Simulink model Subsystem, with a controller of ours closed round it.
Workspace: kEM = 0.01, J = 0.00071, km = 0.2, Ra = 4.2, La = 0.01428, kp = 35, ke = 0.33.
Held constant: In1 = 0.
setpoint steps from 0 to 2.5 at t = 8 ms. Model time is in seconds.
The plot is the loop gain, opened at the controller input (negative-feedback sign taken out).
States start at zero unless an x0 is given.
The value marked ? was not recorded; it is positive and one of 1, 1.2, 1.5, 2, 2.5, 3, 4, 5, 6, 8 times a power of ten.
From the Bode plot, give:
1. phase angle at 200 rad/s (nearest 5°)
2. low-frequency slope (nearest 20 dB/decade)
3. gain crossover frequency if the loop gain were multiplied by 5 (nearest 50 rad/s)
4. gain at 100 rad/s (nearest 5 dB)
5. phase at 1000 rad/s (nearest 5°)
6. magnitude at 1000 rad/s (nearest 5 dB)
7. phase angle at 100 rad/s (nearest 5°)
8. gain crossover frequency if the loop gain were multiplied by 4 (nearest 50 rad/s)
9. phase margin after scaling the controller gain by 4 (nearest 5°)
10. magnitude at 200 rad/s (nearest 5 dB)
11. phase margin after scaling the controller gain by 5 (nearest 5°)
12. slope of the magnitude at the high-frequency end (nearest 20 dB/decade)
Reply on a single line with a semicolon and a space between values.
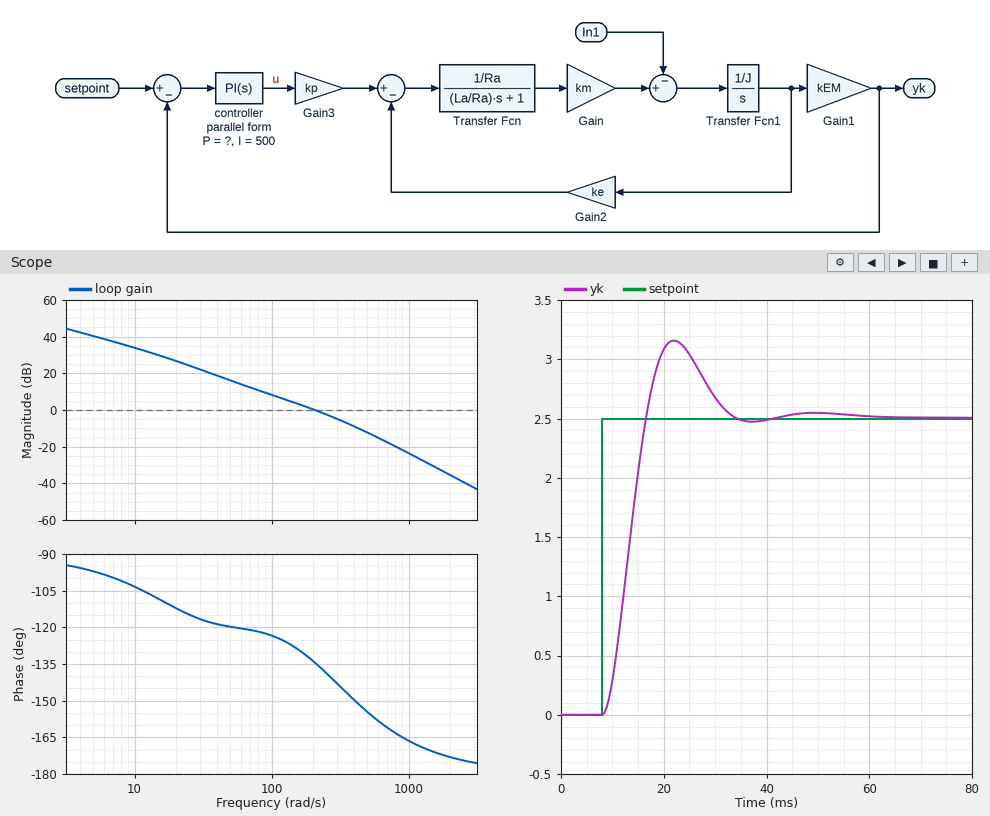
-135°; -20 dB/decade; 550 rad/s; 10 dB; -165°; -25 dB; -125°; 500 rad/s; 25°; 0 dB; 25°; -40 dB/decade
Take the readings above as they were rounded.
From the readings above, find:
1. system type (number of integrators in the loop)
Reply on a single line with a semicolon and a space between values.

1
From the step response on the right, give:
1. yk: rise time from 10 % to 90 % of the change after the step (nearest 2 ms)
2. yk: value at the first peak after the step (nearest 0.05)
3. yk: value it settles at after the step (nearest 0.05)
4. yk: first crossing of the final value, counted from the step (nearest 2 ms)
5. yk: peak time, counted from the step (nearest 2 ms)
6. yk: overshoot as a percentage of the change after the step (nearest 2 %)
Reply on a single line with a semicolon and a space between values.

6 ms; 3.15; 2.50; 8 ms; 14 ms; 26 %
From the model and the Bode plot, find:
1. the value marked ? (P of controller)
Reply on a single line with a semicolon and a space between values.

10
